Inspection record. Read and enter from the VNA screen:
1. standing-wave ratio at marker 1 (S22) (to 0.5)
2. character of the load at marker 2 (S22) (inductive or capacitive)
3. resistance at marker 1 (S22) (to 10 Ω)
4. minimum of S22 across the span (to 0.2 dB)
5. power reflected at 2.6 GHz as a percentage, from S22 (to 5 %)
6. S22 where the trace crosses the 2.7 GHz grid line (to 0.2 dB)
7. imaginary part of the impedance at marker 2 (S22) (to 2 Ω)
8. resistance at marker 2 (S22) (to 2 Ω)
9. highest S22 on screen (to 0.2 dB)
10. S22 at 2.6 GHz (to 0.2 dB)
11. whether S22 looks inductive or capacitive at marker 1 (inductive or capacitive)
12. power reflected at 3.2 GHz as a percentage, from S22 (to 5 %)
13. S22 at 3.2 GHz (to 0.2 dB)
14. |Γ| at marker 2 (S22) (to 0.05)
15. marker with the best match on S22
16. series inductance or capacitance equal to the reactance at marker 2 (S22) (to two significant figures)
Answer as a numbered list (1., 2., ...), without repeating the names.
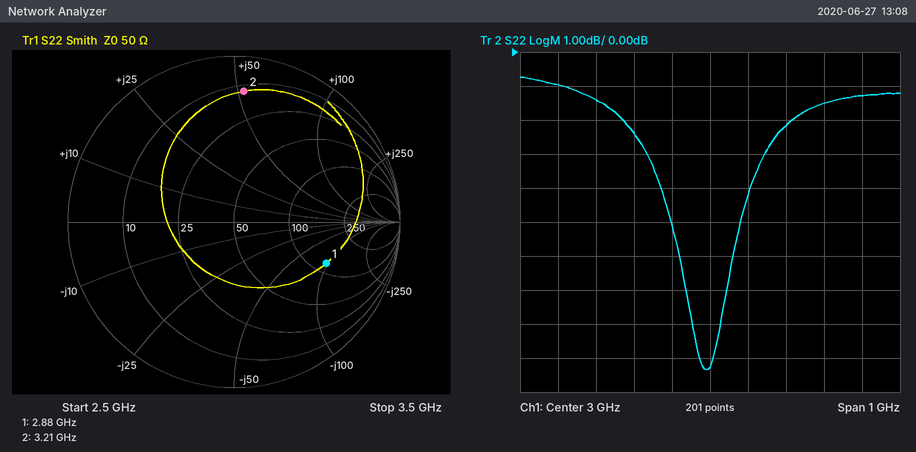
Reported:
1. 4.0
2. inductive
3. 120 Ω
4. -9.4 dB
5. 80 %
6. -1.4 dB
7. +52 Ω
8. 12 Ω
9. -0.8 dB
10. -1.0 dB
11. capacitive
12. 60 %
13. -2.2 dB
14. 0.80
15. marker 1
16. 2.6 nH
